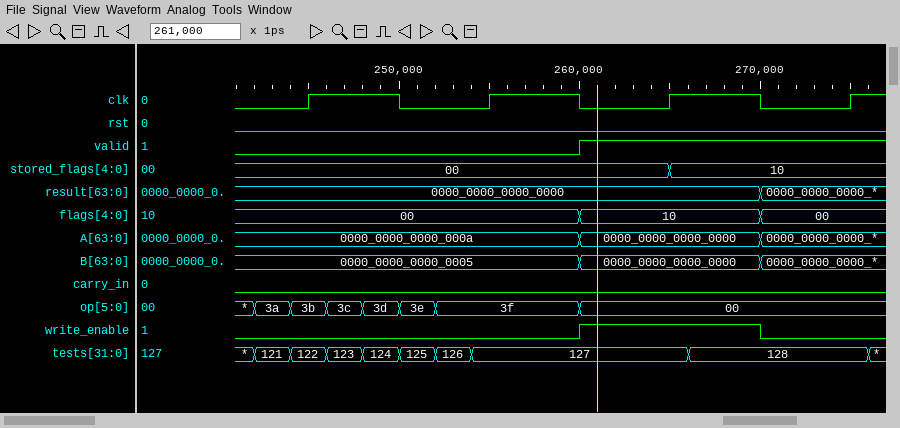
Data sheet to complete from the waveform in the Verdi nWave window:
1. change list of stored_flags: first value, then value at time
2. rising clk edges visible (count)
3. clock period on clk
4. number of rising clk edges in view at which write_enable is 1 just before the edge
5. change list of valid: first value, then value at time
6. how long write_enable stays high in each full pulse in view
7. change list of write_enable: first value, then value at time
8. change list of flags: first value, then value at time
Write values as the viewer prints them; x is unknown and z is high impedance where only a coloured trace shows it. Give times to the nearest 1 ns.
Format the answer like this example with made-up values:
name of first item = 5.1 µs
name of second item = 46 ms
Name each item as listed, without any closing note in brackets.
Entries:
change list of stored_flags: first value, then value at time = 00, 10 at 265 ns
rising clk edges visible = 4
clock period on clk = 10 ns
number of rising clk edges in view at which write_enable is 1 just before the edge = 1
change list of valid: first value, then value at time = 0, 1 at 260 ns
how long write_enable stays high in each full pulse in view = 10 ns
change list of write_enable: first value, then value at time = 0, 1 at 260 ns, 0 at 270 ns
change list of flags: first value, then value at time = 00, 10 at 260 ns, 00 at 270 ns
